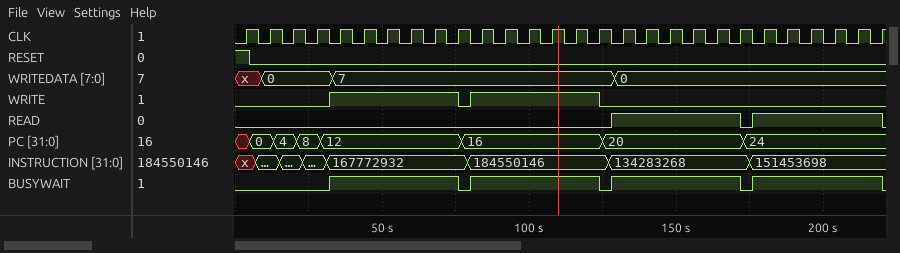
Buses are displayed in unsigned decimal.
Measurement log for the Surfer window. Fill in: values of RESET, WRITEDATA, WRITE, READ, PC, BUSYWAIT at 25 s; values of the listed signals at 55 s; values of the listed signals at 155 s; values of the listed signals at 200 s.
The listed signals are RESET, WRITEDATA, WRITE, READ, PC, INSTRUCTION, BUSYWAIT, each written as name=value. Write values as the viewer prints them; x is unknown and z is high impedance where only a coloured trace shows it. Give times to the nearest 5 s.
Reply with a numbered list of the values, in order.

1. RESET=0, WRITEDATA=0, WRITE=0, READ=0, PC=8, BUSYWAIT=0
2. RESET=0, WRITEDATA=7, WRITE=1, READ=0, PC=12, INSTRUCTION=167772932, BUSYWAIT=1
3. RESET=0, WRITEDATA=0, WRITE=0, READ=1, PC=20, INSTRUCTION=134283268, BUSYWAIT=1
4. RESET=0, WRITEDATA=0, WRITE=0, READ=1, PC=24, INSTRUCTION=151453698, BUSYWAIT=1
